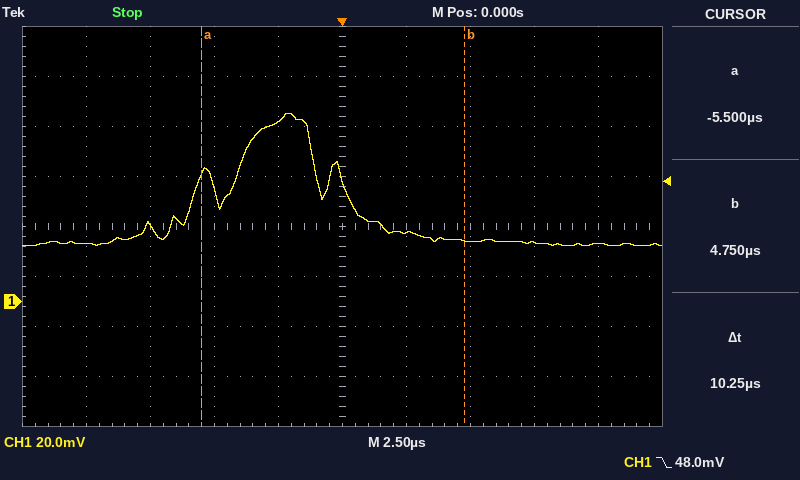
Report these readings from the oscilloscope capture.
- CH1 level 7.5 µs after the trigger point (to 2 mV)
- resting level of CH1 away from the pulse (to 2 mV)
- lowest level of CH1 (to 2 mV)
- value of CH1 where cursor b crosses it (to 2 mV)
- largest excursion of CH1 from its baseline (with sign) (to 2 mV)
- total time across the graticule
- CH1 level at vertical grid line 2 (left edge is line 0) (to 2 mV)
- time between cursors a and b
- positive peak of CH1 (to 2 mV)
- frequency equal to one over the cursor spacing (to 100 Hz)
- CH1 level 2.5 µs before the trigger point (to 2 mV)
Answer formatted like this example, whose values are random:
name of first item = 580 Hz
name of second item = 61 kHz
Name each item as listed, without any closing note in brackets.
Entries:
CH1 level 7.5 µs after the trigger point = 24 mV
resting level of CH1 away from the pulse = 24 mV
lowest level of CH1 = 22 mV
value of CH1 where cursor b crosses it = 24 mV
largest excursion of CH1 from its baseline (with sign) = +52 mV
total time across the graticule = 25 µs
CH1 level at vertical grid line 2 (left edge is line 0) = 30 mV
time between cursors a and b = 10.25 µs
positive peak of CH1 = 76 mV
frequency equal to one over the cursor spacing = 97.6 kHz
CH1 level 2.5 µs before the trigger point = 72 mV
